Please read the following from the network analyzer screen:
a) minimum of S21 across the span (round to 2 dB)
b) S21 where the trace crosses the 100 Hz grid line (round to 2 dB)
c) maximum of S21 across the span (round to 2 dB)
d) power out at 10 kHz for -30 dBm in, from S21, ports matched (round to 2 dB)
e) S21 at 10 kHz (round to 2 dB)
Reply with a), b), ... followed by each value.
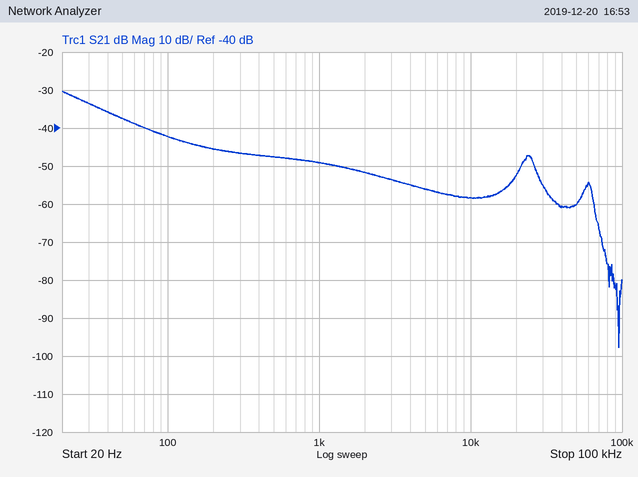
a) -98 dB
b) -42 dB
c) -30 dB
d) -88 dBm
e) -58 dB
